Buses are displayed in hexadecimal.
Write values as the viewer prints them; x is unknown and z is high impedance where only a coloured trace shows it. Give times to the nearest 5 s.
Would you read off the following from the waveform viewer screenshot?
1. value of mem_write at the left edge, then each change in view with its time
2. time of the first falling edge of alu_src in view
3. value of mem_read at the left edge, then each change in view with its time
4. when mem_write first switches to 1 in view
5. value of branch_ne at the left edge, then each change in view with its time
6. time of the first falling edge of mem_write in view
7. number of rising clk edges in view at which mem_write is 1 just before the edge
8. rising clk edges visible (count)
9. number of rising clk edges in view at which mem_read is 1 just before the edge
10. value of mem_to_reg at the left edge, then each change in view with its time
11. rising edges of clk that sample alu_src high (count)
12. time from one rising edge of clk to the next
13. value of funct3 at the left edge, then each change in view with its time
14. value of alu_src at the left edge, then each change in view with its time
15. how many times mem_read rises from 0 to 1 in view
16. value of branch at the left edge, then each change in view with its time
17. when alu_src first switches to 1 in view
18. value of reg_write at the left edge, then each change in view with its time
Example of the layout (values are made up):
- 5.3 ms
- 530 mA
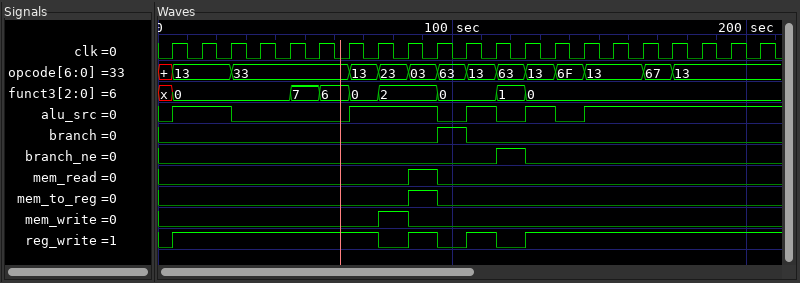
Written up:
- 0, 1 at 75 s, 0 at 85 s
- 25 s
- 0, 1 at 85 s, 0 at 95 s
- 75 s
- 0, 1 at 115 s, 0 at 125 s
- 85 s
- 1
- 21
- 1
- 0, 1 at 85 s, 0 at 95 s
- 13
- 10 s
- x, 0 at 5 s, 7 at 45 s, 6 at 55 s, 0 at 65 s, 2 at 75 s, 0 at 95 s, 1 at 115 s, 0 at 125 s
- 0, 1 at 5 s, 0 at 25 s, 1 at 65 s, 0 at 95 s, 1 at 105 s, 0 at 115 s, 1 at 125 s, 0 at 135 s, 1 at 145 s
- 1
- 0, 1 at 95 s, 0 at 105 s
- 5 s
- 0, 1 at 5 s, 0 at 75 s, 1 at 85 s, 0 at 95 s, 1 at 105 s, 0 at 115 s, 1 at 125 s
